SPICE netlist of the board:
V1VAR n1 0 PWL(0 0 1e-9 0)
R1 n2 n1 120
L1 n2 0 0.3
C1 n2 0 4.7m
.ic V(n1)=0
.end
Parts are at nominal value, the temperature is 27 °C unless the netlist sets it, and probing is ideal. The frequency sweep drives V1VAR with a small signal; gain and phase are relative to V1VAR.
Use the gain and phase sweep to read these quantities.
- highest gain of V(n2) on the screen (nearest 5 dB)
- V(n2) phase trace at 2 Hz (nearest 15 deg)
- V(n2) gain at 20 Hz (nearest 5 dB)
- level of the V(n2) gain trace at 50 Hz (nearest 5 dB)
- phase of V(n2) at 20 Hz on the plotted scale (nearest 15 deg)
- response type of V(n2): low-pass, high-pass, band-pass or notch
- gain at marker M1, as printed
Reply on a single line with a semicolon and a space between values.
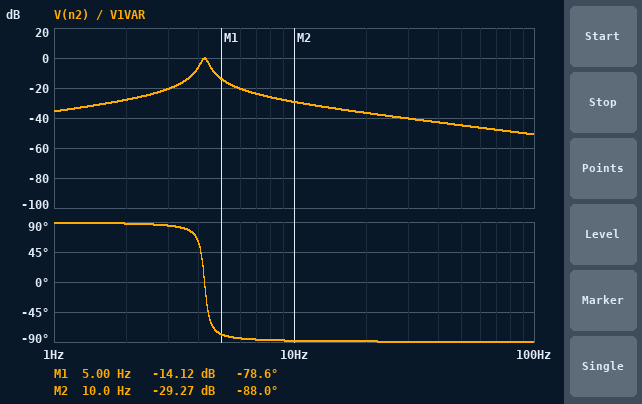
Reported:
0 dB; 90 deg; -35 dB; -45 dB; -90 deg; band-pass; -14.12 dB
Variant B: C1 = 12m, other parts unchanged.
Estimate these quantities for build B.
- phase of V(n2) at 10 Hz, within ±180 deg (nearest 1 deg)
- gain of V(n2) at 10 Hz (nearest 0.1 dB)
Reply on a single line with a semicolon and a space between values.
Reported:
-89 deg; -38.5 dB
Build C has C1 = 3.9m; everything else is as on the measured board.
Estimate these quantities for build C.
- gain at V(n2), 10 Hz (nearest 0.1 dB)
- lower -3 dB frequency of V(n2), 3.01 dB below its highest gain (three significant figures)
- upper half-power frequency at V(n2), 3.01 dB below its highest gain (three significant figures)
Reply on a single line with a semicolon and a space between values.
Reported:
-27.3 dB; 4.49 Hz; 4.83 Hz
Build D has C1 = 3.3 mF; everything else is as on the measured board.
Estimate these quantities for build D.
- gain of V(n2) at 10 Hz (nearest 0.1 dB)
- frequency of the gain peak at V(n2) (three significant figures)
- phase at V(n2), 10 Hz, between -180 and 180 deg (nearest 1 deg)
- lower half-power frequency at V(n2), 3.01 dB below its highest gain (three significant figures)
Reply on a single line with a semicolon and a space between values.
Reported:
-25.4 dB; 5.06 Hz; -87 deg; 4.86 Hz
